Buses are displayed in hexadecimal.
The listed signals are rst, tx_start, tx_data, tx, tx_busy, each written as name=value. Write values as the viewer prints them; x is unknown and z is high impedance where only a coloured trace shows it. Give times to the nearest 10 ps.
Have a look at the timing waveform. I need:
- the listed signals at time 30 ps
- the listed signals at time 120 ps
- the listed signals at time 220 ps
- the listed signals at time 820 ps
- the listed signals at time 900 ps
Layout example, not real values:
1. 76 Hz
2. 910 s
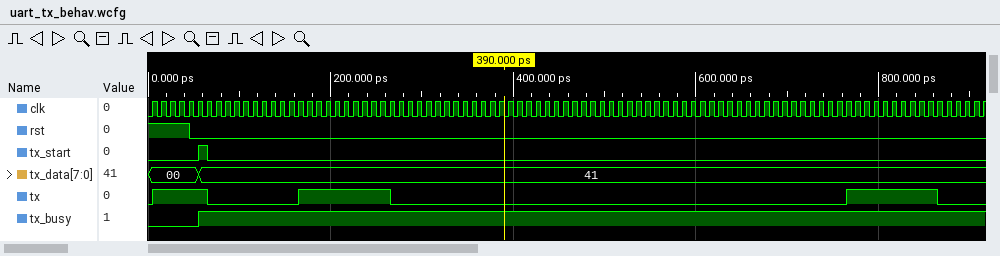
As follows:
1. rst=1, tx_start=0, tx_data=00, tx=1, tx_busy=0
2. rst=0, tx_start=0, tx_data=41, tx=0, tx_busy=1
3. rst=0, tx_start=0, tx_data=41, tx=1, tx_busy=1
4. rst=0, tx_start=0, tx_data=41, tx=1, tx_busy=1
5. rst=0, tx_start=0, tx_data=41, tx=0, tx_busy=1
